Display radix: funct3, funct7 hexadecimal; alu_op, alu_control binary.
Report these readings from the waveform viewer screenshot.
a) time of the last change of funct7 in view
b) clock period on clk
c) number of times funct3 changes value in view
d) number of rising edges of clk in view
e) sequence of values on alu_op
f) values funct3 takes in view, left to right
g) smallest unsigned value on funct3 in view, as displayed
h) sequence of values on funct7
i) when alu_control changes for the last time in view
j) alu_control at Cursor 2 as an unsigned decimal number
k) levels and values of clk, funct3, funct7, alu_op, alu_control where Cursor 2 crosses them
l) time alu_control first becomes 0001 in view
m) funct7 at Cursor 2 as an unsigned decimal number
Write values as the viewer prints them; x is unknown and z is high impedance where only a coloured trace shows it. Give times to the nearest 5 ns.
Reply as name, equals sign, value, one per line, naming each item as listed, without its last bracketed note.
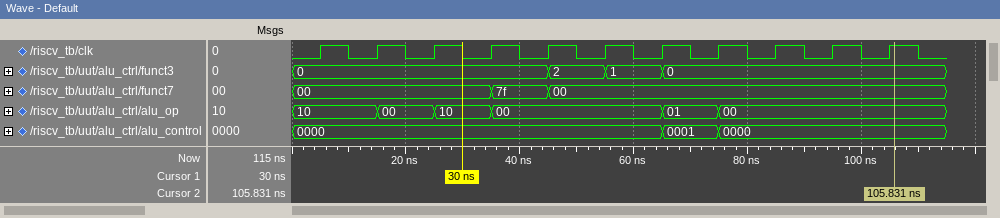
time of the last change of funct7 in view = 45 ns
clock period on clk = 10 ns
number of times funct3 changes value in view = 3
number of rising edges of clk in view = 11
sequence of values on alu_op = 10, 00, 10, 00, 01, 00
values funct3 takes in view, left to right = 0, 2, 1, 0
smallest unsigned value on funct3 in view, as displayed = 0
sequence of values on funct7 = 00, 7f, 00
when alu_control changes for the last time in view = 75 ns
alu_control at Cursor 2 as an unsigned decimal number = 0
levels and values of clk, funct3, funct7, alu_op, alu_control where Cursor 2 crosses them = clk=1, funct3=0, funct7=00, alu_op=00, alu_control=0000
time alu_control first becomes 0001 in view = 65 ns
funct7 at Cursor 2 as an unsigned decimal number = 0
